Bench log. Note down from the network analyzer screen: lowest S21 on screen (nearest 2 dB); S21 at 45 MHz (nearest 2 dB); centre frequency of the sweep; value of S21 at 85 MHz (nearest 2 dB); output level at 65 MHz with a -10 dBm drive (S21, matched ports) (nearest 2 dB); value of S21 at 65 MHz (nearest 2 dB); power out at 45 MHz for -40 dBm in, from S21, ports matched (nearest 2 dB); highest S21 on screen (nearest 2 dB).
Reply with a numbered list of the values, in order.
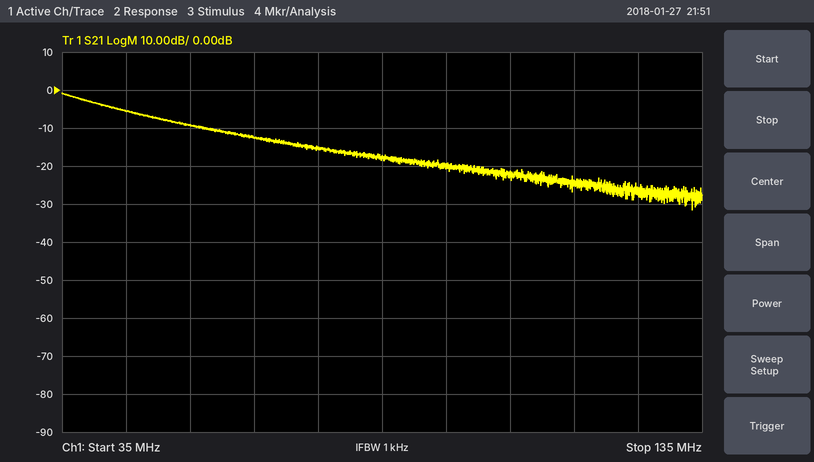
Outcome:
1. -32 dB
2. -6 dB
3. 85 MHz
4. -18 dB
5. -22 dBm
6. -12 dB
7. -46 dBm
8. 0 dB
